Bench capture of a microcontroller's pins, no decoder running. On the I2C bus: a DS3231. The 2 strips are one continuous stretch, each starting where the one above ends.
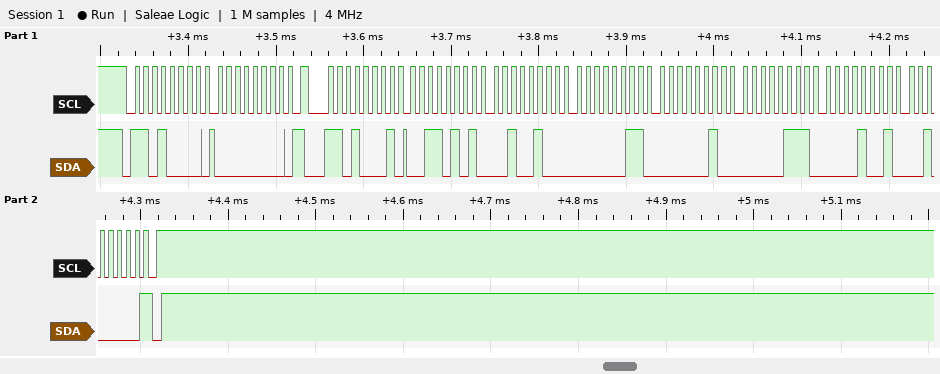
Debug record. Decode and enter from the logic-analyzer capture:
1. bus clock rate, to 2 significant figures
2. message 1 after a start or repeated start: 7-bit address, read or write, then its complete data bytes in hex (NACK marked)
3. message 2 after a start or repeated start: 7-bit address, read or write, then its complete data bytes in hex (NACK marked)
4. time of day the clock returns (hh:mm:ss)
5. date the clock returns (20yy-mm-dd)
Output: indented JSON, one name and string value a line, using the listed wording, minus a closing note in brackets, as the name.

{
  "bus clock rate, to 2 significant figures": "100 kHz",
  "message 1 after a start or repeated start: 7-bit address, read or write, then its complete data bytes in hex": "0x68 write: 00",
  "message 2 after a start or repeated start: 7-bit address, read or write, then its complete data bytes in hex": "0x68 read: 35 24 03 02 07 09 20 NACK",
  "time of day the clock returns": "03:24:35",
  "date the clock returns": "2020-09-07"
}
